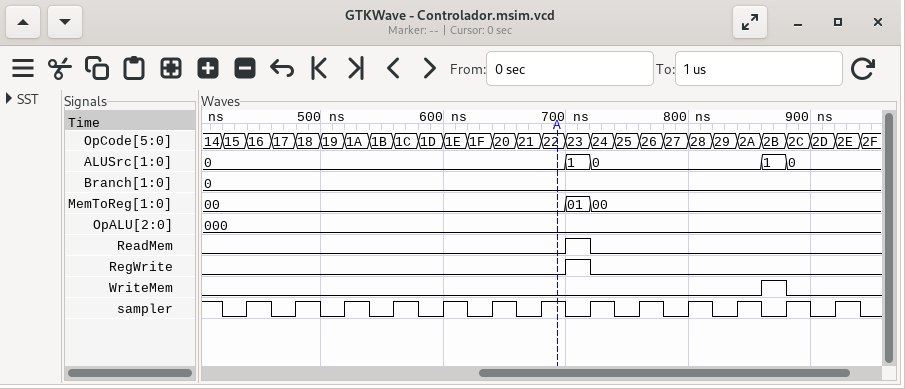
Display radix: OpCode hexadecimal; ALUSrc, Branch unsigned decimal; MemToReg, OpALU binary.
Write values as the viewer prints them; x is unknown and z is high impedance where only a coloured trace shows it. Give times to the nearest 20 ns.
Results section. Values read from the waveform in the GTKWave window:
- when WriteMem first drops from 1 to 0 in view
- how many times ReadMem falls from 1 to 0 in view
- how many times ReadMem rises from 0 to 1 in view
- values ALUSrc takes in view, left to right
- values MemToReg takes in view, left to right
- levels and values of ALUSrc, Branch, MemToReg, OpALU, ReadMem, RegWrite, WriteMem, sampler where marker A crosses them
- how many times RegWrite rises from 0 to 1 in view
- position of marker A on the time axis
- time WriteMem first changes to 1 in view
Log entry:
880 ns
1
1
0, 1, 0, 1, 0
00, 01, 00
ALUSrc=0, Branch=0, MemToReg=00, OpALU=000, ReadMem=0, RegWrite=0, WriteMem=0, sampler=1
1
700 ns
860 ns
